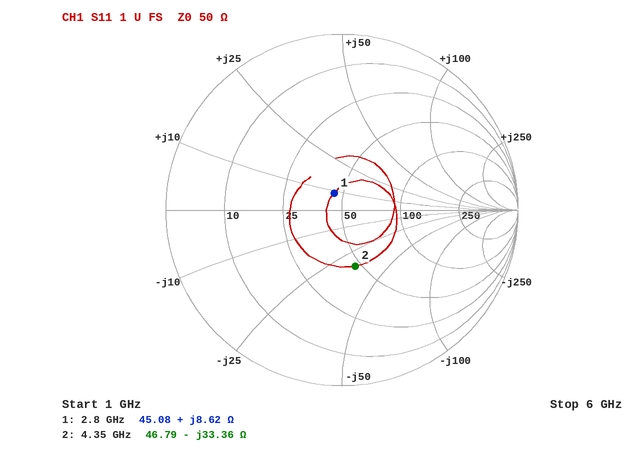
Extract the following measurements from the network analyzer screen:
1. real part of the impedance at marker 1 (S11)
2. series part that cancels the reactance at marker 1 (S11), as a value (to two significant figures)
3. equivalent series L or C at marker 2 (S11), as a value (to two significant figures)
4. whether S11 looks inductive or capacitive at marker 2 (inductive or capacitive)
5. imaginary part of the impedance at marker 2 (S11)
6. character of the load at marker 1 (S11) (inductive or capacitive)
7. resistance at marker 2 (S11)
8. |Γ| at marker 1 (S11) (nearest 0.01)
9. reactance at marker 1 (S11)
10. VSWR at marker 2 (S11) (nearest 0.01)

45.08 Ω
6.6 pF
1.1 pF
capacitive
-33.36 Ω
inductive
46.79 Ω
0.10
+8.62 Ω
1.97
